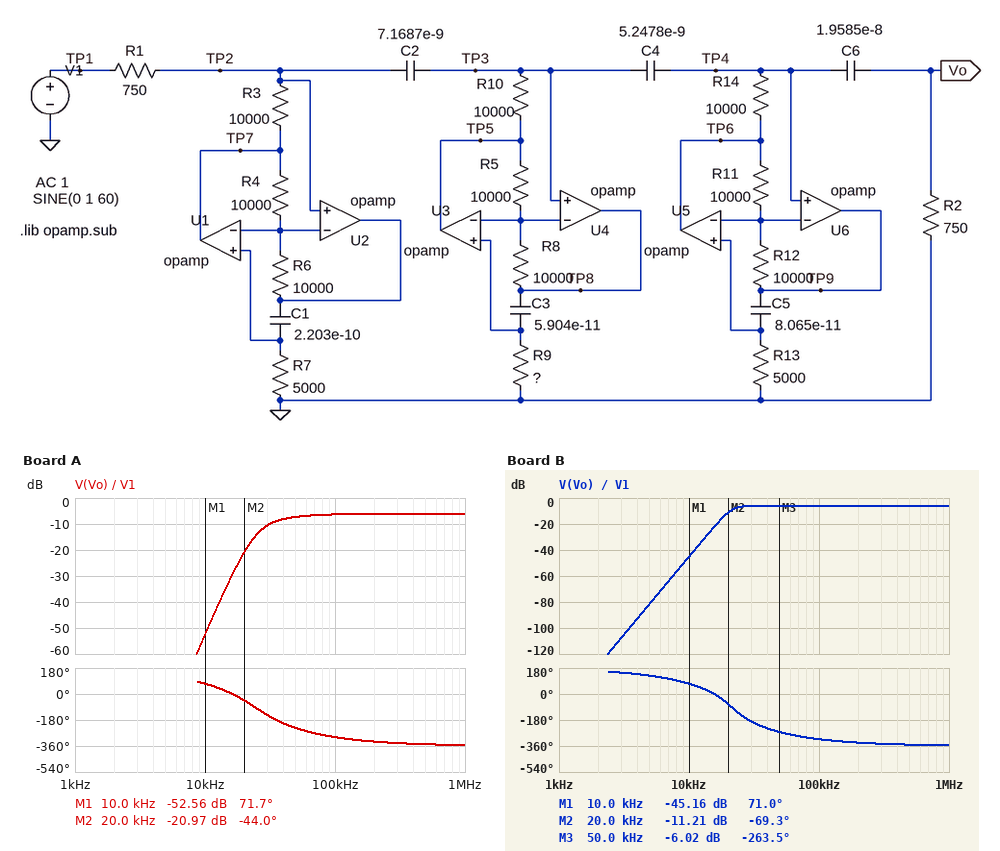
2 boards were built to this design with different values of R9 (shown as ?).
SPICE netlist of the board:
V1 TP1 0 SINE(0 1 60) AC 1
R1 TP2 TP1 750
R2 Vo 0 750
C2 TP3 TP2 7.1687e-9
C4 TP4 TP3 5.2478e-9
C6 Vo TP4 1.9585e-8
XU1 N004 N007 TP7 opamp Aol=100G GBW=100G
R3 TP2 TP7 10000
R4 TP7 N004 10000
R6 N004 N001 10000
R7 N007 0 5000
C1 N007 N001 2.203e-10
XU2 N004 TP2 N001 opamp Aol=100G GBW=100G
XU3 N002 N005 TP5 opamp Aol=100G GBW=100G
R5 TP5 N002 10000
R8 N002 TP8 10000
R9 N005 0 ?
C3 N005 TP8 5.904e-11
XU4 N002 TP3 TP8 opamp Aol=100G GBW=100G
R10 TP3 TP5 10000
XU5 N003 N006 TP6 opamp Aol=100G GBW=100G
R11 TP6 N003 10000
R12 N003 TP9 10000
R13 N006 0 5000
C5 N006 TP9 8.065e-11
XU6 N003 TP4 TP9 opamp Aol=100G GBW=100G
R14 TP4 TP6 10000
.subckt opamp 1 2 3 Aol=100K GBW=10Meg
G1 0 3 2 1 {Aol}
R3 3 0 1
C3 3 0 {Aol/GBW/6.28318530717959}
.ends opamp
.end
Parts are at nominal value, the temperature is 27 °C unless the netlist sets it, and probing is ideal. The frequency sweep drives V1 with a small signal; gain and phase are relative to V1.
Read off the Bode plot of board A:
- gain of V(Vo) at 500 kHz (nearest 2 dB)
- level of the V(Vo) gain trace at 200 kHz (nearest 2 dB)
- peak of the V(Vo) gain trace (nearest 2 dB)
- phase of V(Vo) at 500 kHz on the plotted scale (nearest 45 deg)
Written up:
-6 dB
-6 dB
-6 dB
-360 deg
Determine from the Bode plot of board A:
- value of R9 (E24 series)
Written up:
2.2 kΩ
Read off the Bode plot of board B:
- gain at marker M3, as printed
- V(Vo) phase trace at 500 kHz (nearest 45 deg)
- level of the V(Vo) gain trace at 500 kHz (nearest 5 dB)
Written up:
-6.02 dB
-360 deg
-5 dB
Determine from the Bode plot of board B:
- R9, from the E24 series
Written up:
4.7 kΩ
